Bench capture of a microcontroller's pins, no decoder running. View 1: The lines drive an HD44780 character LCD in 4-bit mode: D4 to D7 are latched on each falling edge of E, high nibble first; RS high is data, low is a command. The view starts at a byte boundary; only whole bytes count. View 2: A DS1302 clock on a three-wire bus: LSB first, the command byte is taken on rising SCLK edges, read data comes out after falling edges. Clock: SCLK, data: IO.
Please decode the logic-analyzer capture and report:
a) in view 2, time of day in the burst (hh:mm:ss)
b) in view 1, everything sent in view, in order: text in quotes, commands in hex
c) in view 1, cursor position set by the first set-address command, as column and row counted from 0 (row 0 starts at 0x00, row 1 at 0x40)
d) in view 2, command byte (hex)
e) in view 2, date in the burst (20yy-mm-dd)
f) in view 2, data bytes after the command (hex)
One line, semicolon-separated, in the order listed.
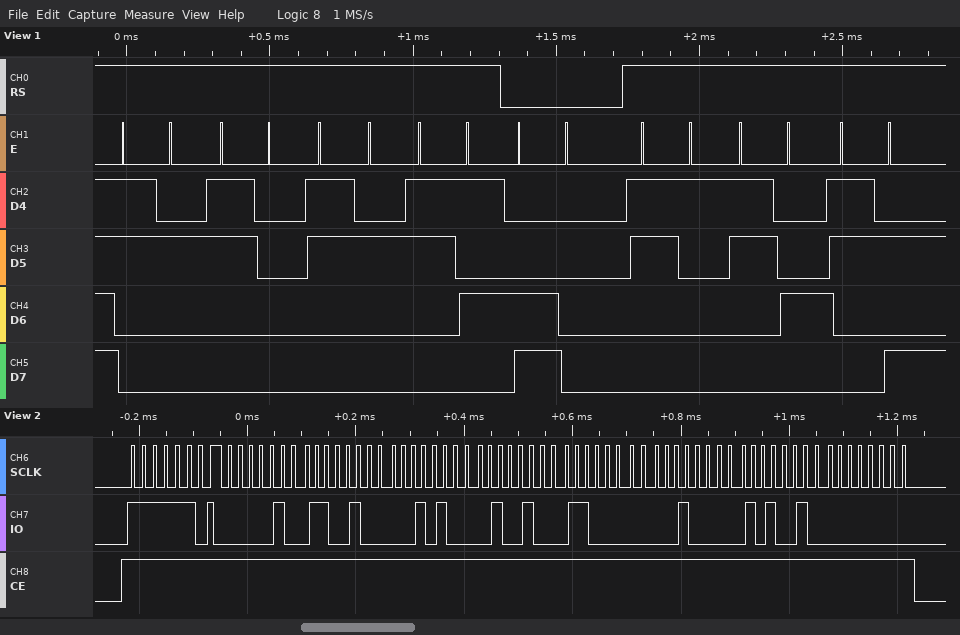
14:13:20; "2025" 0xC0 "14:"; column 0, row 1; 0xBF; 2025-03-12; 20 13 14 12 03 04 25 00
